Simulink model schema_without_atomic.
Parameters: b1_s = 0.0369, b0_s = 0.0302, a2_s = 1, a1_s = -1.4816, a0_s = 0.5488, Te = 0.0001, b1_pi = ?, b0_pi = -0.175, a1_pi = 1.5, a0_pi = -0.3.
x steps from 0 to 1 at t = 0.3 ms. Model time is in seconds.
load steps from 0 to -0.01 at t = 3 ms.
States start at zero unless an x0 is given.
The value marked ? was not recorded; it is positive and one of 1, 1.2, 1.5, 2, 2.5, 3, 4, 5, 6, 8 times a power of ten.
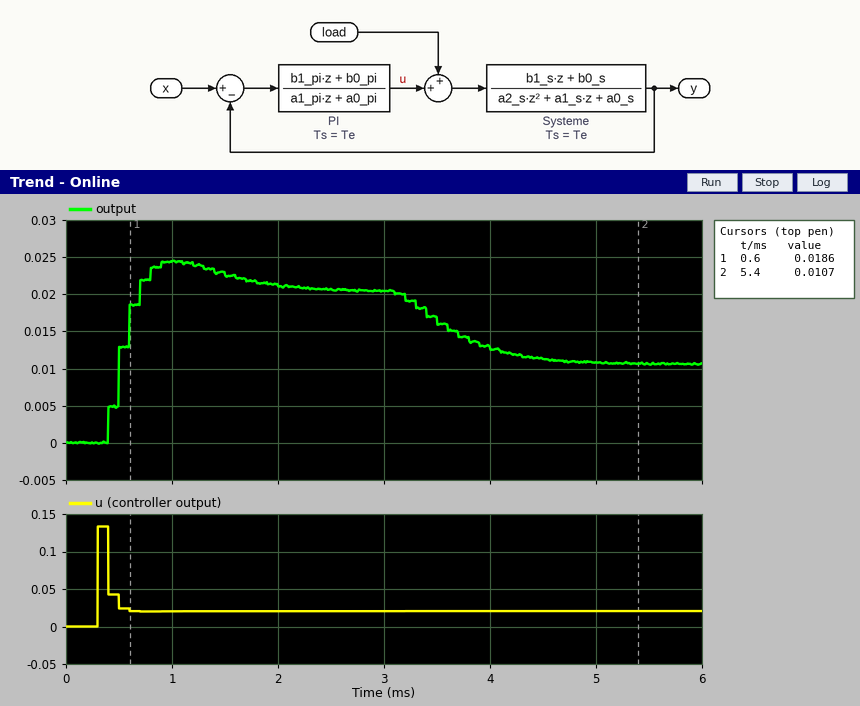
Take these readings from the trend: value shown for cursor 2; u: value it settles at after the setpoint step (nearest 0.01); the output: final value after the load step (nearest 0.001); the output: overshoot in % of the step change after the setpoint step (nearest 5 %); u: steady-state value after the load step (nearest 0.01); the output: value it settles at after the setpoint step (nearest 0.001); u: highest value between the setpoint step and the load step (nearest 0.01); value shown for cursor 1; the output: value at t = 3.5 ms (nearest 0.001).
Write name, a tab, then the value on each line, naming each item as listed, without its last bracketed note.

value shown for cursor 2	0.0107
u: value it settles at after the setpoint step	0.02
the output: final value after the load step	0.011
the output: overshoot in % of the step change after the setpoint step	20 %
u: steady-state value after the load step	0.02
the output: value it settles at after the setpoint step	0.020
u: highest value between the setpoint step and the load step	0.13
value shown for cursor 1	0.0186
the output: value at t = 3.5 ms	0.016
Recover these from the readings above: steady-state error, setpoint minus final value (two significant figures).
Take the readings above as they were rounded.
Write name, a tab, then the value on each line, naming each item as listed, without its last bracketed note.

steady-state error, setpoint minus final value	0.98
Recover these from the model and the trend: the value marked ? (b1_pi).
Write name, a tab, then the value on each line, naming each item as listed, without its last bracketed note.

the value marked ?	0.2
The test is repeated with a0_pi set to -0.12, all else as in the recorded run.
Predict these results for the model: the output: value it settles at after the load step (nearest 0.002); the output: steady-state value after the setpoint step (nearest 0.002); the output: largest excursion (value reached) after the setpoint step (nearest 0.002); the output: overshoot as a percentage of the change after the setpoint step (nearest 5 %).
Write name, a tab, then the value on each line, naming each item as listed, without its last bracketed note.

the output: value it settles at after the load step	0.008
the output: steady-state value after the setpoint step	0.018
the output: largest excursion (value reached) after the setpoint step	0.022
the output: overshoot as a percentage of the change after the setpoint step	20 %
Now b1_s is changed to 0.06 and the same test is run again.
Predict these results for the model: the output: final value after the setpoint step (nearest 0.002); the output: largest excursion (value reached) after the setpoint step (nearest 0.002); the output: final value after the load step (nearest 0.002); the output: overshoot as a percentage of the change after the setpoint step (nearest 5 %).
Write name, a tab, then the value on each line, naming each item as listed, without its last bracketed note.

the output: final value after the setpoint step	0.028
the output: largest excursion (value reached) after the setpoint step	0.032
the output: final value after the load step	0.014
the output: overshoot as a percentage of the change after the setpoint step	20 %
